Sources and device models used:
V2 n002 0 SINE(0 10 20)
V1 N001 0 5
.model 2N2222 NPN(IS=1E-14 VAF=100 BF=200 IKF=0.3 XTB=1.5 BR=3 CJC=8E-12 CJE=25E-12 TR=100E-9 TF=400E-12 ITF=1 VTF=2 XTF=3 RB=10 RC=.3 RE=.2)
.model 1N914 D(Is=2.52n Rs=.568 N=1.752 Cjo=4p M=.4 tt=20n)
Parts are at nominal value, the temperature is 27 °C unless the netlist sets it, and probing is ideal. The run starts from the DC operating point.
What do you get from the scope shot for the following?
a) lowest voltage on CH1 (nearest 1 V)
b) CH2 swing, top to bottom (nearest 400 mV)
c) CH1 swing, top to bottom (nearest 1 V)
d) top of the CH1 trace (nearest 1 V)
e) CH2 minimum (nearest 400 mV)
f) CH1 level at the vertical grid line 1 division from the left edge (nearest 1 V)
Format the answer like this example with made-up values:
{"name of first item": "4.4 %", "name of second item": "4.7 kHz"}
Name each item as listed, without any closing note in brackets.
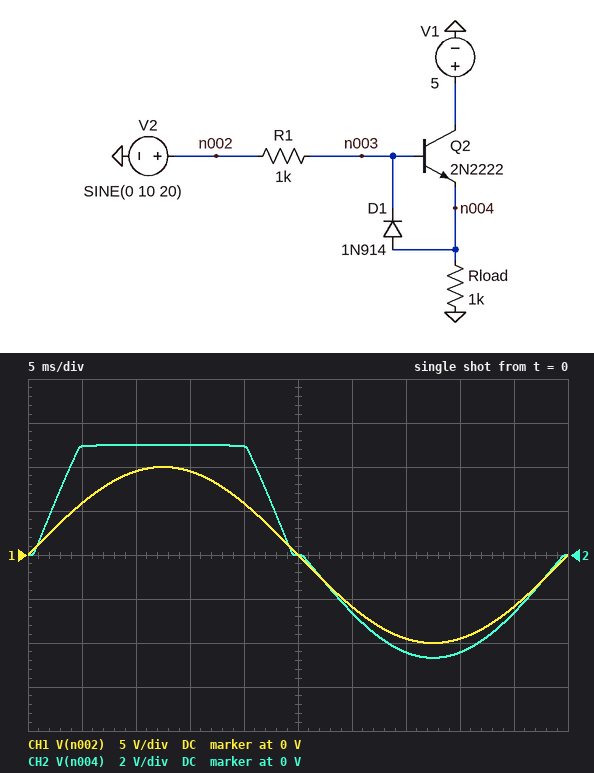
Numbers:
{"lowest voltage on CH1": "-10 V", "CH2 swing, top to bottom": "9.6 V", "CH1 swing, top to bottom": "20 V", "top of the CH1 trace": "10 V", "CH2 minimum": "-4.8 V", "CH1 level at the vertical grid line 1 division from the left edge": "6 V"}
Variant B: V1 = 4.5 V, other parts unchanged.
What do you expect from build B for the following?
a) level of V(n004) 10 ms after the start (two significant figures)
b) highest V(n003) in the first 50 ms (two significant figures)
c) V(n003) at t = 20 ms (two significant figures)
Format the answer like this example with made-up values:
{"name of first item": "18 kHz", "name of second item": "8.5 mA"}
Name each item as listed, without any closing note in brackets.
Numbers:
{"level of V(n004) 10 ms after the start": "4.5 V", "highest V(n003) in the first 50 ms": "5.3 V", "V(n003) at t = 20 ms": "5.2 V"}
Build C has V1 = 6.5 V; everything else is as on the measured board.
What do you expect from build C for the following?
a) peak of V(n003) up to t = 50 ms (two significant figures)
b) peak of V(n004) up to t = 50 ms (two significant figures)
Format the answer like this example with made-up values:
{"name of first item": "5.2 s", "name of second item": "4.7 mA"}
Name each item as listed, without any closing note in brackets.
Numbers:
{"peak of V(n003) up to t = 50 ms": "7.2 V", "peak of V(n004) up to t = 50 ms": "6.5 V"}
